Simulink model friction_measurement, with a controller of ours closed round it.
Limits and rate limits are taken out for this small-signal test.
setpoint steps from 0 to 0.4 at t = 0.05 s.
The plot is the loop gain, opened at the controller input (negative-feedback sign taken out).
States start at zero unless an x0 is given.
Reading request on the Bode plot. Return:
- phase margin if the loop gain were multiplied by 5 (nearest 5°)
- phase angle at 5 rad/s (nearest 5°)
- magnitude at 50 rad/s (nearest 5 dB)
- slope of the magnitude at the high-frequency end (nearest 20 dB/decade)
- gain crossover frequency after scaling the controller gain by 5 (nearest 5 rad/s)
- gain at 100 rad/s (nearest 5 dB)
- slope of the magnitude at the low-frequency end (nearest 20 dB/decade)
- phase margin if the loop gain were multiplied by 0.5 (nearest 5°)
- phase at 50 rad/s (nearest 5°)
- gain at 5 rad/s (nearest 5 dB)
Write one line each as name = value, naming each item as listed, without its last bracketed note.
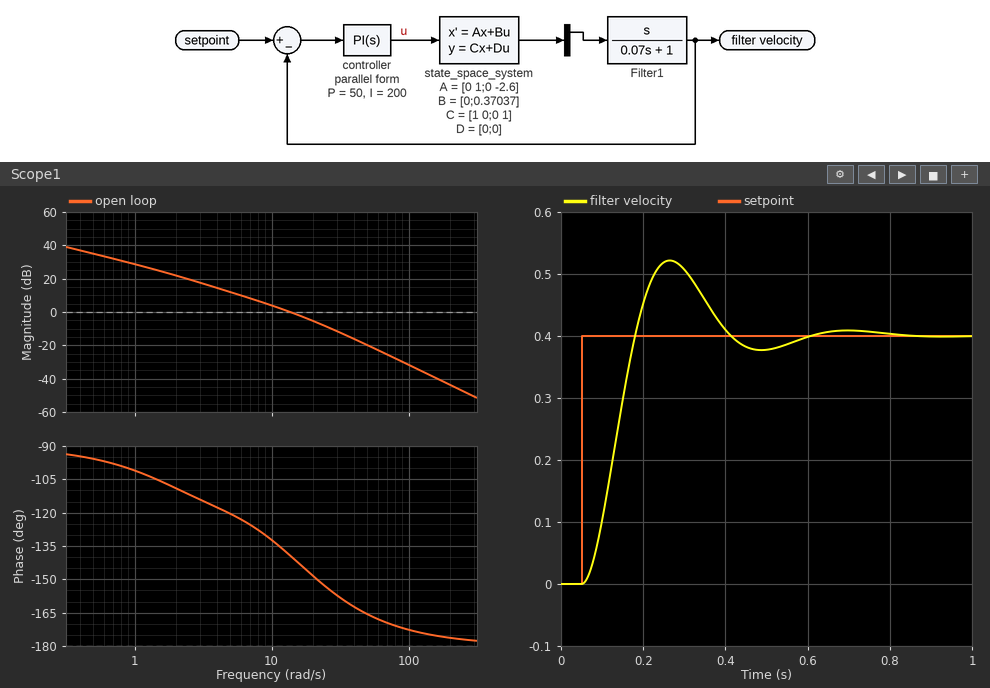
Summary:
phase margin if the loop gain were multiplied by 5 = 20°
phase angle at 5 rad/s = -120°
magnitude at 50 rad/s = -20 dB
slope of the magnitude at the high-frequency end = -40 dB/decade
gain crossover frequency after scaling the controller gain by 5 = 35 rad/s
gain at 100 rad/s = -30 dB
slope of the magnitude at the low-frequency end = -20 dB/decade
phase margin if the loop gain were multiplied by 0.5 = 50°
phase at 50 rad/s = -165°
gain at 5 rad/s = 10 dB
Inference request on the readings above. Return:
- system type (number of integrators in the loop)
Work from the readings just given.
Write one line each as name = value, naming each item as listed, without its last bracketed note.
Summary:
system type = 1
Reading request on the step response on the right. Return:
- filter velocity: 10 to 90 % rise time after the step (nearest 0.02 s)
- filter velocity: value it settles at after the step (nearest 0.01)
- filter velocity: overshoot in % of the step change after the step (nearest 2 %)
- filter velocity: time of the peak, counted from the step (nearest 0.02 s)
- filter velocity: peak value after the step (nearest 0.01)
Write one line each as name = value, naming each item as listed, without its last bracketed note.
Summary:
filter velocity: 10 to 90 % rise time after the step = 0.08 s
filter velocity: value it settles at after the step = 0.40
filter velocity: overshoot in % of the step change after the step = 30 %
filter velocity: time of the peak, counted from the step = 0.22 s
filter velocity: peak value after the step = 0.52
